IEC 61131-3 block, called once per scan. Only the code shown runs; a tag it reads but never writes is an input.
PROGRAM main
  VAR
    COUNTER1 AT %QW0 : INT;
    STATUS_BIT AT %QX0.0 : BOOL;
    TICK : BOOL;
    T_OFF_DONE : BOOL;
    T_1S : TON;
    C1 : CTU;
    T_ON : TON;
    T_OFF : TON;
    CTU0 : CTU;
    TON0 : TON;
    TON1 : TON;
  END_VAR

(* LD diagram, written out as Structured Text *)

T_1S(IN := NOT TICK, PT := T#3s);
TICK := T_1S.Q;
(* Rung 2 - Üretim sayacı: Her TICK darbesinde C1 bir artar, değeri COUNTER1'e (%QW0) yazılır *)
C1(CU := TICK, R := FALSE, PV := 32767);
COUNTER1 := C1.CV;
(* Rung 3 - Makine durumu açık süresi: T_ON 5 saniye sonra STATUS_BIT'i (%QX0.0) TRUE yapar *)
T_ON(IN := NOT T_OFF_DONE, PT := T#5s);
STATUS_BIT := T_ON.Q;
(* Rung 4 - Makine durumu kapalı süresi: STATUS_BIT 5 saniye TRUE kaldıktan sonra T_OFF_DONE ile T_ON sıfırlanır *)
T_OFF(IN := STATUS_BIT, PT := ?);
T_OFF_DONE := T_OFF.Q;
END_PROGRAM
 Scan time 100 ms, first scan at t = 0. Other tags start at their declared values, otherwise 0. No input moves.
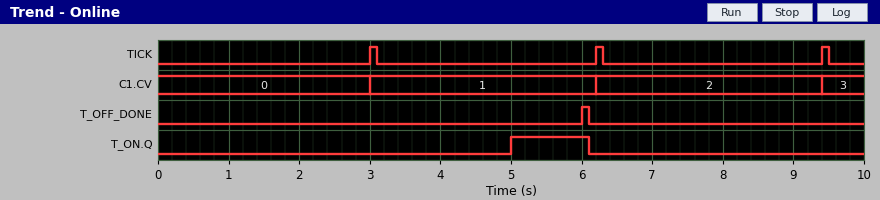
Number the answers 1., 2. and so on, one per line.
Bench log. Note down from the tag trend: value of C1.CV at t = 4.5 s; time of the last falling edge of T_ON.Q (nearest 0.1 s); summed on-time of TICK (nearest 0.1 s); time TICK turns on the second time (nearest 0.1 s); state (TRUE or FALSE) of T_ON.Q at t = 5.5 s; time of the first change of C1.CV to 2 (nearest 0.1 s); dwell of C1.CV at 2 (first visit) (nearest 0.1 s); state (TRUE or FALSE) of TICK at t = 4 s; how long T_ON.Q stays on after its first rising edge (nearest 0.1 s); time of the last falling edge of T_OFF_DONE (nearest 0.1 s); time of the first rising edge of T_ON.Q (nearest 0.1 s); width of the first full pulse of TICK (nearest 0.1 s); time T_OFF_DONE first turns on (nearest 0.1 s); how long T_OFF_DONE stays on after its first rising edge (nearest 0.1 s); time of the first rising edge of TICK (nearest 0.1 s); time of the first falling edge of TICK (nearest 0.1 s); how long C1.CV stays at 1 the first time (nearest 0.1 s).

1. 1
2. 6.1 s
3. 0.3 s
4. 6.2 s
5. TRUE
6. 6.2 s
7. 3.2 s
8. FALSE
9. 1.1 s
10. 6.1 s
11. 5.0 s
12. 0.1 s
13. 6.0 s
14. 0.1 s
15. 3.0 s
16. 3.1 s
17. 3.2 s
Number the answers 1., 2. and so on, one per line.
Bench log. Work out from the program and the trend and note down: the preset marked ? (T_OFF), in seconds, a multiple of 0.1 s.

1. 1.0 s
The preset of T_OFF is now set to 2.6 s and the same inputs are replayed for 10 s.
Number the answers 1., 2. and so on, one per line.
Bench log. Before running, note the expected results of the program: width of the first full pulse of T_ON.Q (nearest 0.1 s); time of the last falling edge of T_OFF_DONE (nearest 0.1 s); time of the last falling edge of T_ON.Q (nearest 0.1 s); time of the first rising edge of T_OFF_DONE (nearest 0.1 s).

1. 2.7 s
2. 7.7 s
3. 7.7 s
4. 7.6 s
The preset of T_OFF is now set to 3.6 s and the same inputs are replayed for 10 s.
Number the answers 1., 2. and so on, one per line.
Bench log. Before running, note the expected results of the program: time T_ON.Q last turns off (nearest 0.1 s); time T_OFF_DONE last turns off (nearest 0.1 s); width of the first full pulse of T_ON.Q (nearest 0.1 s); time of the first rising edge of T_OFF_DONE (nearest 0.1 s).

1. 8.7 s
2. 8.7 s
3. 3.7 s
4. 8.6 s
